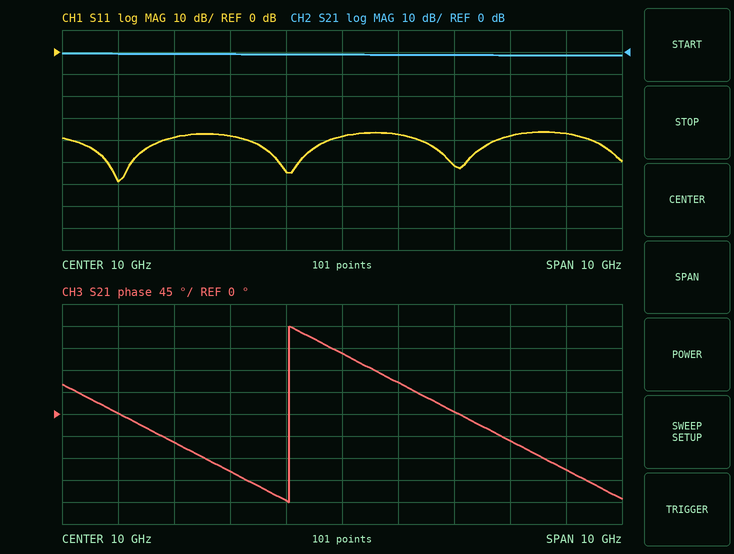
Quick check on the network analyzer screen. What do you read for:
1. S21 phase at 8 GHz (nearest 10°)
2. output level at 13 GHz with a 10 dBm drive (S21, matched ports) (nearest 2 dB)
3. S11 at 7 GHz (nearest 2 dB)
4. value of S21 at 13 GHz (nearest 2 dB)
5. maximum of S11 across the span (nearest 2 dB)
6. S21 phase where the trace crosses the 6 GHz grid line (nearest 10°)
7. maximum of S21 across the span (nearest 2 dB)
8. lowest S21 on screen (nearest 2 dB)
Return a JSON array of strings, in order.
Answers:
["-120°", "8 dBm", "-38 dB", "-2 dB", "-36 dB", "0°", "0 dB", "-2 dB"]
